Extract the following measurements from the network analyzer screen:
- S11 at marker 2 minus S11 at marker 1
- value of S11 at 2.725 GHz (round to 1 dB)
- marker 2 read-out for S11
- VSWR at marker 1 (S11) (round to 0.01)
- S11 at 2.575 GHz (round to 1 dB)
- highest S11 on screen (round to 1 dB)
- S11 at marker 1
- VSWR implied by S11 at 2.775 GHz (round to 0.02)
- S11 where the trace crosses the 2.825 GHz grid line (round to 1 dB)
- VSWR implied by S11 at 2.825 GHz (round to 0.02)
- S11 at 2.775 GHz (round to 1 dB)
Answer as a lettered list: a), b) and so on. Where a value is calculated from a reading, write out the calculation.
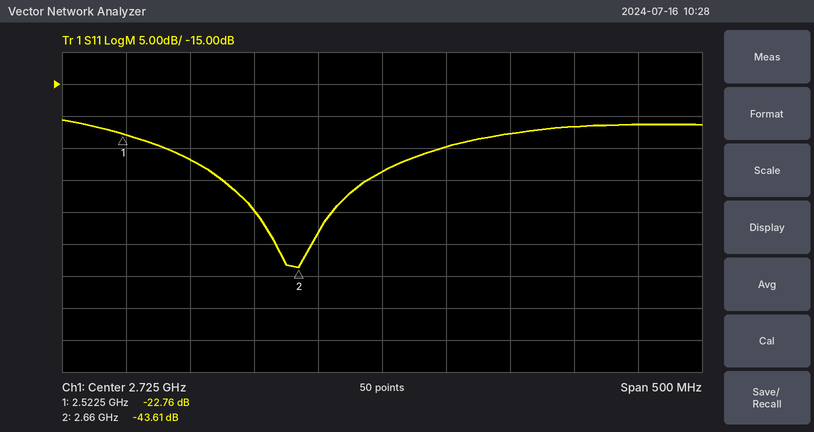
a) -43.61 − (-22.76) = -20.85 dB
b) -29 dB
c) -43.61 dB
d) (1 + 0.0728)/(1 − 0.0728) ≈ 1.16
e) -27 dB
f) -21 dB
g) -22.76 dB
h) |Γ| = 10^(-25/20) = 0.0562; VSWR = (1 + 0.0562)/(1 − 0.0562) ≈ 1.12
i) -23 dB
j) |Γ| = 10^(-23/20) = 0.0708; VSWR = (1 + 0.0708)/(1 − 0.0708) ≈ 1.15, so 1.16 to the nearest 0.02
k) -25 dB
